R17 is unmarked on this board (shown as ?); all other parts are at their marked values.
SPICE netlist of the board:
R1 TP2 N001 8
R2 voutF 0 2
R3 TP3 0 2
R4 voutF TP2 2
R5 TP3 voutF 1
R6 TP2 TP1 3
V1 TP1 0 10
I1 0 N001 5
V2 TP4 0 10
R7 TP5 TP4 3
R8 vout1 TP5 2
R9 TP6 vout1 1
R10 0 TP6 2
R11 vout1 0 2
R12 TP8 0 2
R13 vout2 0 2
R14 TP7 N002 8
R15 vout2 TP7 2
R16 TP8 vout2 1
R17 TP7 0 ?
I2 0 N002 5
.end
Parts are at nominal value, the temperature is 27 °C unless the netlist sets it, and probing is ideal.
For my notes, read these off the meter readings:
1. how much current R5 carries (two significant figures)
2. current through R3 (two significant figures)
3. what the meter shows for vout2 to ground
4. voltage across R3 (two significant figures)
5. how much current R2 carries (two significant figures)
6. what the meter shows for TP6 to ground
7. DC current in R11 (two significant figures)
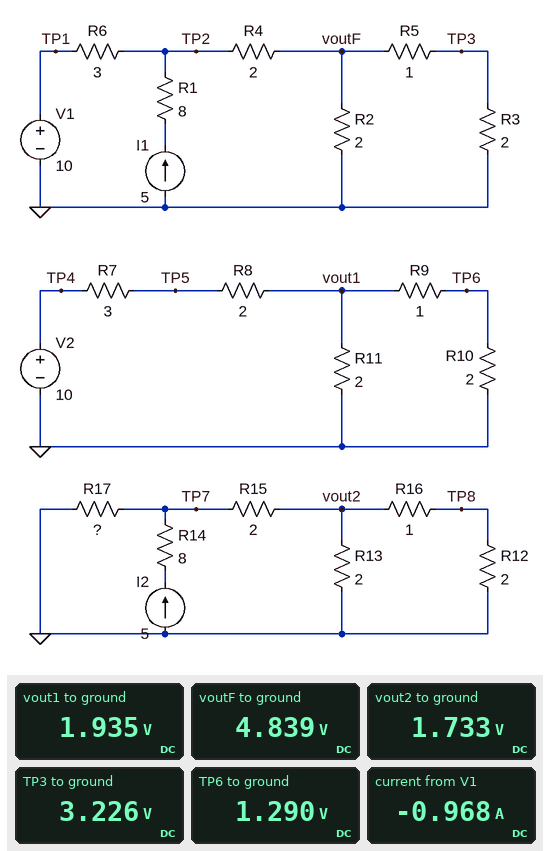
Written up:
1.6 A
1.6 A
1.733 V
3.2 V
2.4 A
1.290 V
970 mA
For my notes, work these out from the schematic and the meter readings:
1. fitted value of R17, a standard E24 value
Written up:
1.3 Ω
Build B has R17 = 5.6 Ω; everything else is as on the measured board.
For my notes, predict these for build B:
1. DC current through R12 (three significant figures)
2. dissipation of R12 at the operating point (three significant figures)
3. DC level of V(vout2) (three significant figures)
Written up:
1.27 A
3.24 W
3.82 V
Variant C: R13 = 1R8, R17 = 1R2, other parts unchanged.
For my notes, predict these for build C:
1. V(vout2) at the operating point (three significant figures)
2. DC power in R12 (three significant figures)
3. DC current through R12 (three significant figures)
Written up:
1.56 V
541 mW
520 mA
